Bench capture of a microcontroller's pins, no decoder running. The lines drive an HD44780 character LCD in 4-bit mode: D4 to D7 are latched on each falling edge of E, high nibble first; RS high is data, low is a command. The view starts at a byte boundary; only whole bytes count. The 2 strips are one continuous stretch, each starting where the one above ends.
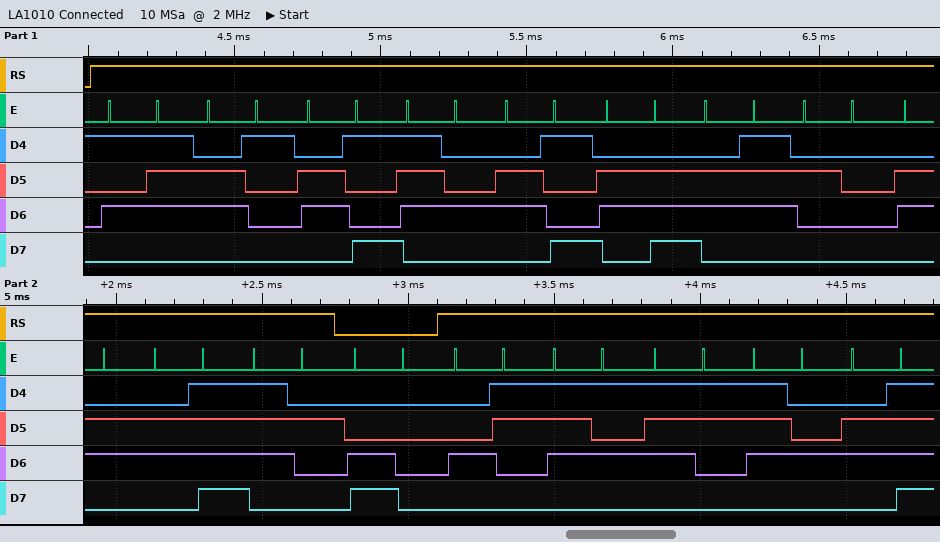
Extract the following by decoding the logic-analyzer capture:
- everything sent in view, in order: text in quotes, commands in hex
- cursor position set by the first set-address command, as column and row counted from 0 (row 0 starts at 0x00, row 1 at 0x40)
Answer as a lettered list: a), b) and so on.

a) "Waiting for" 0xC0 "Custo"
b) column 0, row 1
